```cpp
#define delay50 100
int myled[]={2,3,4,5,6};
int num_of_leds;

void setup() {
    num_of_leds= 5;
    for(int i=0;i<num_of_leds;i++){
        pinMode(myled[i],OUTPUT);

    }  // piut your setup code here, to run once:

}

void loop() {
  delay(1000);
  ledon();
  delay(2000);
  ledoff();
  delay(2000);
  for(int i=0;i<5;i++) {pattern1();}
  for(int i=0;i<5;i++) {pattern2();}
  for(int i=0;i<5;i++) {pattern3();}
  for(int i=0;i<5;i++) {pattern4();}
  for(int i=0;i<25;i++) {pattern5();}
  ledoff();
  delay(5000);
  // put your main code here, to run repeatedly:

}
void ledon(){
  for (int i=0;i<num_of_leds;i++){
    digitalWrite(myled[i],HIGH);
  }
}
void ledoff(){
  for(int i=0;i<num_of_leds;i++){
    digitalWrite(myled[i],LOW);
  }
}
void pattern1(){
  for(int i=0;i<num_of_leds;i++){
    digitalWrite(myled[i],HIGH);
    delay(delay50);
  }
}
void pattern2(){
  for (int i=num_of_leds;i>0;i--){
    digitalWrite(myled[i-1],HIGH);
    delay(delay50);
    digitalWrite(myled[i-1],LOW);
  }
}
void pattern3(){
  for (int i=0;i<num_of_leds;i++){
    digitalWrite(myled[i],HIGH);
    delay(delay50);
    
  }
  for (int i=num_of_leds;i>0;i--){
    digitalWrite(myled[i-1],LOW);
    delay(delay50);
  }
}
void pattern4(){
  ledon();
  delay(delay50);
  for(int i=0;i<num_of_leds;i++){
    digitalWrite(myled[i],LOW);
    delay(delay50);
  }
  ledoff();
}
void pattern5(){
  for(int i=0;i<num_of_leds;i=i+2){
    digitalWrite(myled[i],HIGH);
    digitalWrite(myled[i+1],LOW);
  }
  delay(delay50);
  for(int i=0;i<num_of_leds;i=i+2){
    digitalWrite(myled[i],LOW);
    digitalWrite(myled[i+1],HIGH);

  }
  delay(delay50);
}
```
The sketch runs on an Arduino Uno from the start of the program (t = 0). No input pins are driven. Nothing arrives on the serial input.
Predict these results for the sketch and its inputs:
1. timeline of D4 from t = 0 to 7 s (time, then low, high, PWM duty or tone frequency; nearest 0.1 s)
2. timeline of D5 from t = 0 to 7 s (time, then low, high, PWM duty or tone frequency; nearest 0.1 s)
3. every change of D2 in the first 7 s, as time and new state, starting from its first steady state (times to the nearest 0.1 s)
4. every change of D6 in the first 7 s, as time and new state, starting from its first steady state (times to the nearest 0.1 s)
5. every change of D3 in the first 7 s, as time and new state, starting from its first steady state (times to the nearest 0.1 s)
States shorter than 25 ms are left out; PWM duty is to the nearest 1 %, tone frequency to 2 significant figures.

0 s low; 1 s high; 3 s low; 5.2 s high
0 s low; 1 s high; 3 s low; 5.3 s high
0 s low; 1 s high; 3 s low; 5 s high
0 s low; 1 s high; 3 s low; 5.4 s high
0 s low; 1 s high; 3 s low; 5.1 s high
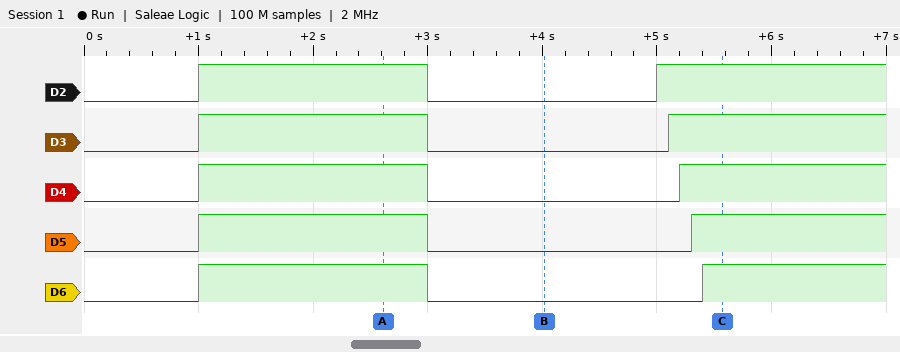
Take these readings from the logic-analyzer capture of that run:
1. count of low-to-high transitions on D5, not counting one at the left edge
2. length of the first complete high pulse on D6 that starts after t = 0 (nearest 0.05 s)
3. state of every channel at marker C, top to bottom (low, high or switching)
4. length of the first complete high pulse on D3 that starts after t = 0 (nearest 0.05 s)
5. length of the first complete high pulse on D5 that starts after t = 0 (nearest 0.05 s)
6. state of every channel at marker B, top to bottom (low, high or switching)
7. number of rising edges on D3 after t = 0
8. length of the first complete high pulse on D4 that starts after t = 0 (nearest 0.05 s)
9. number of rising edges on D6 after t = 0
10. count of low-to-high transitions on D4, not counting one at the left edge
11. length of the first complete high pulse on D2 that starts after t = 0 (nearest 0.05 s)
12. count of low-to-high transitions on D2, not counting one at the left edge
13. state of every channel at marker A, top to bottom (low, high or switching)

2
2.00 s
D2 high, D3 high, D4 high, D5 high, D6 high
2.00 s
2.00 s
D2 low, D3 low, D4 low, D5 low, D6 low
2
2.00 s
2
2
2.00 s
2
D2 high, D3 high, D4 high, D5 high, D6 high
